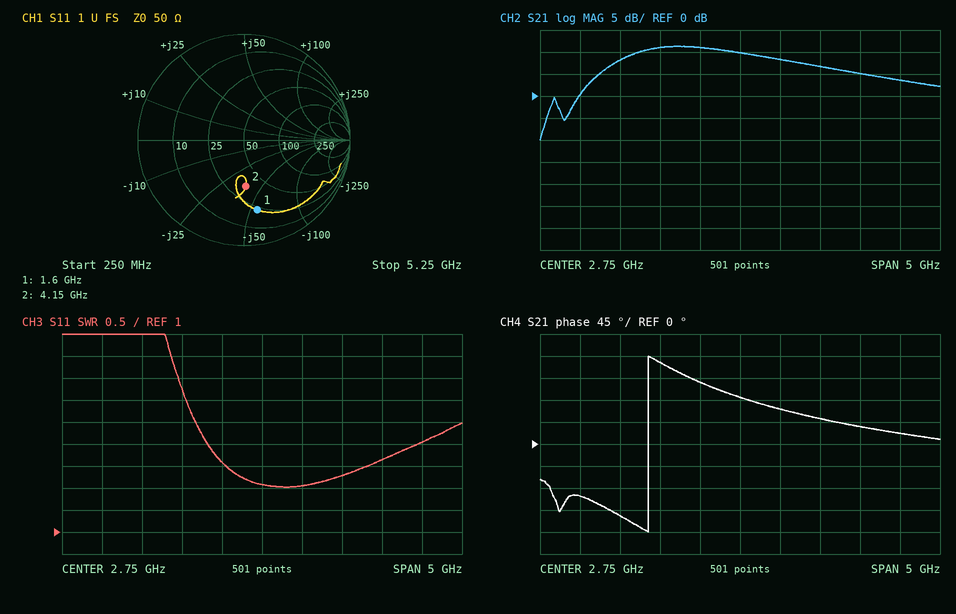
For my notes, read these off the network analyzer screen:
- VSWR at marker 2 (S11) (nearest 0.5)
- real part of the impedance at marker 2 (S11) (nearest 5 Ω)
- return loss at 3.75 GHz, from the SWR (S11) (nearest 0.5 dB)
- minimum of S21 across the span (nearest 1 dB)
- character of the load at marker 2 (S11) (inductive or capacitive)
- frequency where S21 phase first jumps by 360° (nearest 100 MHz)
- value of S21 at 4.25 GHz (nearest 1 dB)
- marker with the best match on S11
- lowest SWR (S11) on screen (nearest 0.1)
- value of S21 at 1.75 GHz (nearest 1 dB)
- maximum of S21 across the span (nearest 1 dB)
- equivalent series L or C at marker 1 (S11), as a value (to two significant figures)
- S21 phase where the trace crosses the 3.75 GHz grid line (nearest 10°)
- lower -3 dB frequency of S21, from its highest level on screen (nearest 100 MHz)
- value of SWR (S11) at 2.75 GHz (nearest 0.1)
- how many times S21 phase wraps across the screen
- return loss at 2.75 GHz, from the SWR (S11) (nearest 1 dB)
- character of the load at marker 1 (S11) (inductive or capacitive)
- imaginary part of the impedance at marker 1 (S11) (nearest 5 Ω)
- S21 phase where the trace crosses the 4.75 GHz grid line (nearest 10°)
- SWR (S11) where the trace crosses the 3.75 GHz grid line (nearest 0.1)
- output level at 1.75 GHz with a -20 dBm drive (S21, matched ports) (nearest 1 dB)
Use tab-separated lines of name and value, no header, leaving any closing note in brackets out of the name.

VSWR at marker 2 (S11)	2.5
real part of the impedance at marker 2 (S11)	35 Ω
return loss at 3.75 GHz, from the SWR (S11)	8.0 dB
minimum of S21 across the span	-10 dB
character of the load at marker 2 (S11)	capacitive
frequency where S21 phase first jumps by 360°	1.6 GHz
value of S21 at 4.25 GHz	5 dB
marker with the best match on S11	marker 2
lowest SWR (S11) on screen	2.0
value of S21 at 1.75 GHz	11 dB
maximum of S21 across the span	11 dB
equivalent series L or C at marker 1 (S11), as a value	1.8 pF
S21 phase where the trace crosses the 3.75 GHz grid line	50°
lower -3 dB frequency of S21, from its highest level on screen	1.3 GHz
value of SWR (S11) at 2.75 GHz	2.1
how many times S21 phase wraps across the screen	1
return loss at 2.75 GHz, from the SWR (S11)	9 dB
character of the load at marker 1 (S11)	capacitive
imaginary part of the impedance at marker 1 (S11)	-55 Ω
S21 phase where the trace crosses the 4.75 GHz grid line	20°
SWR (S11) where the trace crosses the 3.75 GHz grid line	2.3
output level at 1.75 GHz with a -20 dBm drive (S21, matched ports)	-9 dBm
